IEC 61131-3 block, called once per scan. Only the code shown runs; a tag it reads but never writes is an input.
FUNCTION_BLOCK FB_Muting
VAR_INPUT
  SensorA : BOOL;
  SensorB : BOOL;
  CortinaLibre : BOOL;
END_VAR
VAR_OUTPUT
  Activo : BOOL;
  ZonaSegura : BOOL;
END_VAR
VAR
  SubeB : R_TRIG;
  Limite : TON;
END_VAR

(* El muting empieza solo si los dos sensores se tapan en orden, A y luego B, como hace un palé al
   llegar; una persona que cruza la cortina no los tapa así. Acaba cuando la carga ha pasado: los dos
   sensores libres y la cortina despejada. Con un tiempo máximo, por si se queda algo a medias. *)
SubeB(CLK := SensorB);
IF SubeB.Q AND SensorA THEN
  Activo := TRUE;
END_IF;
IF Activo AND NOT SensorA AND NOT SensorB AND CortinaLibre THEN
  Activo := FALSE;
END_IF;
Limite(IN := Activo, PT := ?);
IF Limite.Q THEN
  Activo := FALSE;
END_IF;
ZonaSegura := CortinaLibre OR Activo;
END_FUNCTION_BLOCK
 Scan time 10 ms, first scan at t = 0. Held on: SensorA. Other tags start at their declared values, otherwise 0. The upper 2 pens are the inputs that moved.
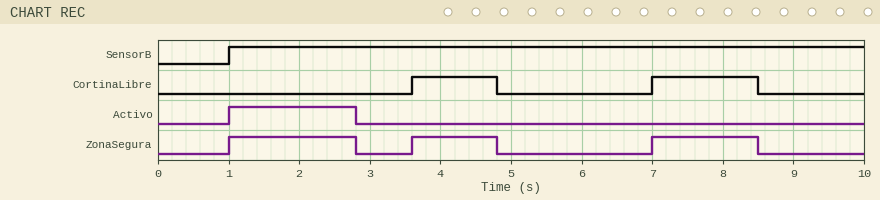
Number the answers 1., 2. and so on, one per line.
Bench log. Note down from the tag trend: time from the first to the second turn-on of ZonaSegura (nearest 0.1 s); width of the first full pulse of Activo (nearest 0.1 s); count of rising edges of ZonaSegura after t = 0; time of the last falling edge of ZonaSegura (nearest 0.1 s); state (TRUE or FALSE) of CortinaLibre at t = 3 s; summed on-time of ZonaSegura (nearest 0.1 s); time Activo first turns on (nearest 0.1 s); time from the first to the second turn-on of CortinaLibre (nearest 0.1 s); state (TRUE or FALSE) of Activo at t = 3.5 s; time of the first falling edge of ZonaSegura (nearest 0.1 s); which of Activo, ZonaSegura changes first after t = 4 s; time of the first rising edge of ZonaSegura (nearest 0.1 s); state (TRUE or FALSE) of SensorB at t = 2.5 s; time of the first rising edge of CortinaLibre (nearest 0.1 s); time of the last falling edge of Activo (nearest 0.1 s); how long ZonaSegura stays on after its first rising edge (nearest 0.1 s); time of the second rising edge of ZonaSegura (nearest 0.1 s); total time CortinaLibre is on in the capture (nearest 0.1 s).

1. 2.6 s
2. 1.8 s
3. 3
4. 8.5 s
5. FALSE
6. 4.5 s
7. 1.0 s
8. 3.4 s
9. FALSE
10. 2.8 s
11. ZonaSegura
12. 1.0 s
13. TRUE
14. 3.6 s
15. 2.8 s
16. 1.8 s
17. 3.6 s
18. 2.7 s
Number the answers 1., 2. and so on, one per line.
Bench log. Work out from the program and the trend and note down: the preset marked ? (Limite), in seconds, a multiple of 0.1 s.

1. 1.8 s
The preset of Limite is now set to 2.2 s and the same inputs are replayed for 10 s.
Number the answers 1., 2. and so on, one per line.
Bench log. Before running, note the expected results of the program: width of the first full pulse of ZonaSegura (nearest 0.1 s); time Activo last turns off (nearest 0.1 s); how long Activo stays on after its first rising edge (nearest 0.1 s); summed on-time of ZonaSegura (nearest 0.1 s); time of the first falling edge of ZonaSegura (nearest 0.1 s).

1. 2.2 s
2. 3.2 s
3. 2.2 s
4. 4.9 s
5. 3.2 s
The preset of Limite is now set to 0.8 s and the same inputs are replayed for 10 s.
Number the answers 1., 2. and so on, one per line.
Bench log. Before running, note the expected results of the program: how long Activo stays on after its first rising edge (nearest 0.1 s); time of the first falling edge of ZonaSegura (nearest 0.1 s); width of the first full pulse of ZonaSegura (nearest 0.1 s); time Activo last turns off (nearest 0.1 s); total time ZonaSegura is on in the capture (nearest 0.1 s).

1. 0.8 s
2. 1.8 s
3. 0.8 s
4. 1.8 s
5. 3.5 s
